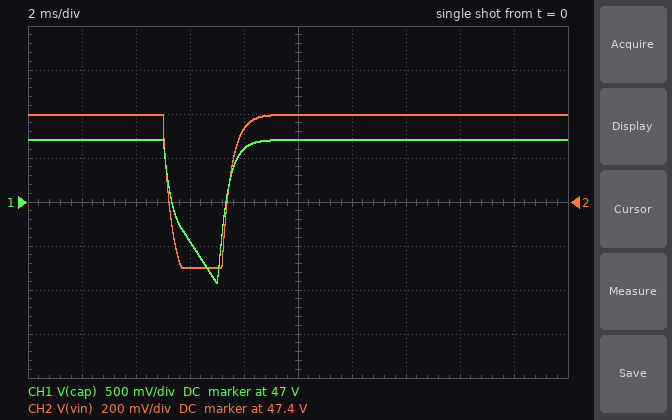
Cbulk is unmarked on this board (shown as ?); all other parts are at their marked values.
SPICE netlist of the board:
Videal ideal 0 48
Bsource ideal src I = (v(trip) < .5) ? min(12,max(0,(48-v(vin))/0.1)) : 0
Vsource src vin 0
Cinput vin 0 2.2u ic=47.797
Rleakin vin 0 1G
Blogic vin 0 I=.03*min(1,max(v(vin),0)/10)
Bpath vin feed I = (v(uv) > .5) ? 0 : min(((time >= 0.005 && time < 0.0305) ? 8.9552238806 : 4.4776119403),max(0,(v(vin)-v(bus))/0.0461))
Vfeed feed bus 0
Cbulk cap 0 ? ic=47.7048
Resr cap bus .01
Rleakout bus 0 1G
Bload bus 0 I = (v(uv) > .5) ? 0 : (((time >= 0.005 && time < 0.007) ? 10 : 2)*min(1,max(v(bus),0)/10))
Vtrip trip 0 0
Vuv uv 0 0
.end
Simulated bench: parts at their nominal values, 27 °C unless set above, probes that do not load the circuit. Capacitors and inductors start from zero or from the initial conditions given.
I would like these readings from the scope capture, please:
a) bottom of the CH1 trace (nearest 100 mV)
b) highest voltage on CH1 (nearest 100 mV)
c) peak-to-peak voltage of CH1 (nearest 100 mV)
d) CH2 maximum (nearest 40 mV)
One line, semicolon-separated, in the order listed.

46.1 V; 47.7 V; 1.6 V; 47.80 V
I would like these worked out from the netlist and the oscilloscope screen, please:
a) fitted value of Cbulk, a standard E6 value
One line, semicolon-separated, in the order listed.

2.2 mF
